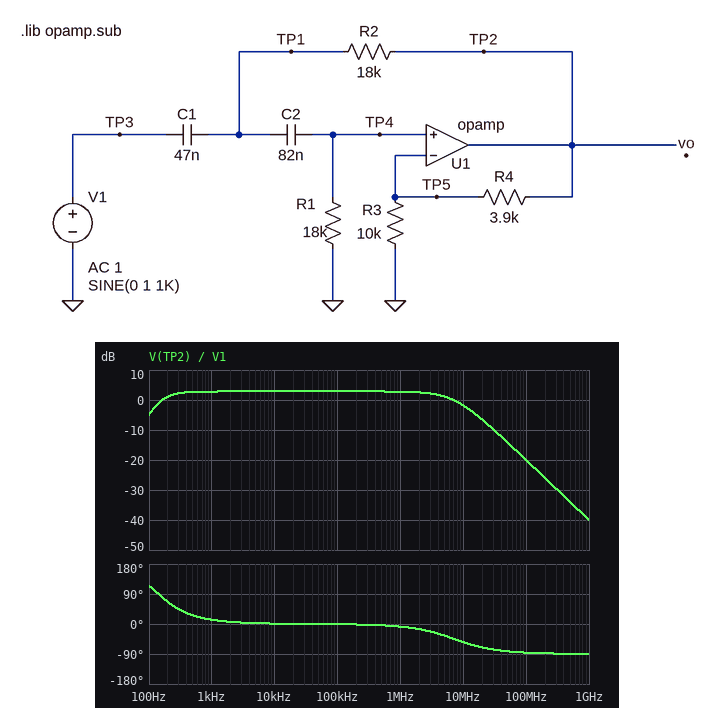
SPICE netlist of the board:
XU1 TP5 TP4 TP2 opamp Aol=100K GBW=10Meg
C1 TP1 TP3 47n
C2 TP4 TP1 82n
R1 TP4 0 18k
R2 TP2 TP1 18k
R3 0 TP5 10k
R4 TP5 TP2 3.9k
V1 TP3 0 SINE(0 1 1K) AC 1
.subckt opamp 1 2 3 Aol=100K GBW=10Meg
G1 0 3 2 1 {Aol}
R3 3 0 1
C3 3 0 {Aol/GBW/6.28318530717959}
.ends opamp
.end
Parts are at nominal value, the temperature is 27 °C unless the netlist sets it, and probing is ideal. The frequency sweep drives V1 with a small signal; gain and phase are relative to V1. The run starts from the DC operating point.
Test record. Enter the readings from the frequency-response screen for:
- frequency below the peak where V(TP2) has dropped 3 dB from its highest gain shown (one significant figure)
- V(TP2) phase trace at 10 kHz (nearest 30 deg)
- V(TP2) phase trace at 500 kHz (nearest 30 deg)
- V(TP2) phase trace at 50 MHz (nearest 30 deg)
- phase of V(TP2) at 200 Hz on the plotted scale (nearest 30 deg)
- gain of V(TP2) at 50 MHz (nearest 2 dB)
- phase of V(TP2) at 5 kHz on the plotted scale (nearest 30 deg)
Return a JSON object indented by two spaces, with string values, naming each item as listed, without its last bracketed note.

{
  "frequency below the peak where V(TP2) has dropped 3 dB from its highest gain shown": "200 Hz",
  "V(TP2) phase trace at 10 kHz": "0 deg",
  "V(TP2) phase trace at 500 kHz": "0 deg",
  "V(TP2) phase trace at 50 MHz": "-90 deg",
  "phase of V(TP2) at 200 Hz on the plotted scale": "60 deg",
  "gain of V(TP2) at 50 MHz": "-14 dB",
  "phase of V(TP2) at 5 kHz on the plotted scale": "0 deg"
}
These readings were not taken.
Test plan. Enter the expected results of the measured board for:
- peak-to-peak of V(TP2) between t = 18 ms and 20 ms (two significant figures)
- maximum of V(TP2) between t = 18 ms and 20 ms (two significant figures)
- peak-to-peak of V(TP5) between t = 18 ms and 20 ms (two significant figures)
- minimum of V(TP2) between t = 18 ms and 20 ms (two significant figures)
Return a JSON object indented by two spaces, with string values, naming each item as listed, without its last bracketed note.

{
  "peak-to-peak of V(TP2) between t = 18 ms and 20 ms": "2.8 V",
  "maximum of V(TP2) between t = 18 ms and 20 ms": "1.4 V",
  "peak-to-peak of V(TP5) between t = 18 ms and 20 ms": "2.0 V",
  "minimum of V(TP2) between t = 18 ms and 20 ms": "-1.4 V"
}
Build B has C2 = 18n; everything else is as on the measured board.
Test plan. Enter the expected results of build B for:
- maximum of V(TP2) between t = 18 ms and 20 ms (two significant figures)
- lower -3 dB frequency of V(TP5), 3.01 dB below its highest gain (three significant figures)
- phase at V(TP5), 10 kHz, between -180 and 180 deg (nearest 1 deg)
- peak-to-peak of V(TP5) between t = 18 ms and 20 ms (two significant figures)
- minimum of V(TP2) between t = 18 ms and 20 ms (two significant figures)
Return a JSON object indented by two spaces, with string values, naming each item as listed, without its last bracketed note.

{
  "maximum of V(TP2) between t = 18 ms and 20 ms": "1.3 V",
  "lower -3 dB frequency of V(TP5), 3.01 dB below its highest gain": "470 Hz",
  "phase at V(TP5), 10 kHz, between -180 and 180 deg": "3 deg",
  "peak-to-peak of V(TP5) between t = 18 ms and 20 ms": "1.8 V",
  "minimum of V(TP2) between t = 18 ms and 20 ms": "-1.3 V"
}
